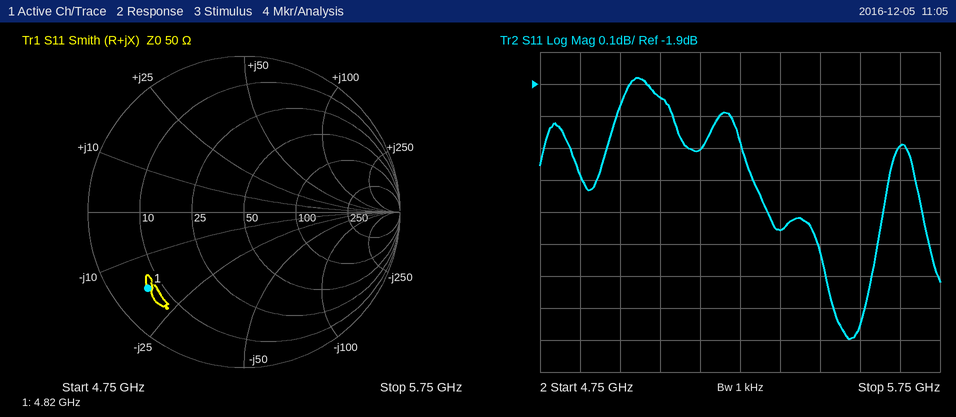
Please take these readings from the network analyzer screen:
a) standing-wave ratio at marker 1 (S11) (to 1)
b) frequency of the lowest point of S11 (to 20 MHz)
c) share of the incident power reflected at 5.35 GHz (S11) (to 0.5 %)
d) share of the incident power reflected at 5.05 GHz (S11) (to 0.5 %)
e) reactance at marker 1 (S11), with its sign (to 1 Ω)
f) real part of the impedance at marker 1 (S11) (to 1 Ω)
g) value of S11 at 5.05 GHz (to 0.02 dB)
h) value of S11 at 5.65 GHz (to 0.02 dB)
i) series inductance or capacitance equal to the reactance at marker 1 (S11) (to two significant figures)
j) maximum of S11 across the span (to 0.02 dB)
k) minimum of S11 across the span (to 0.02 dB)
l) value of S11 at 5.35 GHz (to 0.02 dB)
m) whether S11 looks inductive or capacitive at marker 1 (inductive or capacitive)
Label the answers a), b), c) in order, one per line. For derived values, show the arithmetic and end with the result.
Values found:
a) 8
b) 5.52 GHz
c) 10^(-2.36/10) ≈ 58.1 %, so 58.0 % to the nearest 0.5 %
d) 10^(-1.94/10) ≈ 64.0 %
e) -17 Ω
f) 7 Ω
g) -1.94 dB
h) -2.10 dB
i) C = 1/(2π × 4.82 GHz × 17 Ω) ≈ 1.9 pF
j) -1.88 dB
k) -2.70 dB
l) -2.36 dB
m) capacitive
